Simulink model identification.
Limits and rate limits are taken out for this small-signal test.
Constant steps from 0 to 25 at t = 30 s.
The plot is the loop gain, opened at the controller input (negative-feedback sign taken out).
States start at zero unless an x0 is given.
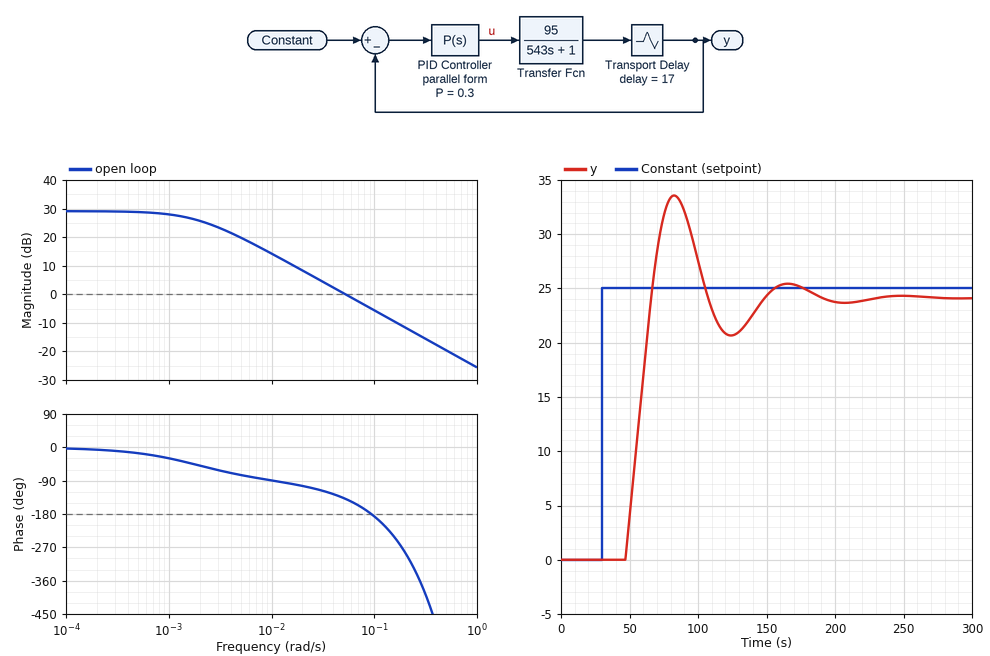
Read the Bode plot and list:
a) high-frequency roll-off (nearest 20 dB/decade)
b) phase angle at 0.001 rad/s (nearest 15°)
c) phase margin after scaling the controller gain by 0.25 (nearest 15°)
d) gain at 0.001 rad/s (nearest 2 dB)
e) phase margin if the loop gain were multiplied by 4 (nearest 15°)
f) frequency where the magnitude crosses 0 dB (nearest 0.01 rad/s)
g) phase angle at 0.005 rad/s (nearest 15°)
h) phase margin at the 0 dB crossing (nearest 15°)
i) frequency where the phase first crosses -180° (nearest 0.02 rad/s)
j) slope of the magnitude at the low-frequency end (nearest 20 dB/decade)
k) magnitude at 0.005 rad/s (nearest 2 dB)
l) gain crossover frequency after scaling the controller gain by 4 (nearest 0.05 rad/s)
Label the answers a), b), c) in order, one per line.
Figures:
a) -20 dB/decade
b) -30°
c) 90°
d) 28 dB
e) -120°
f) 0.05 rad/s
g) -75°
h) 45°
i) 0.10 rad/s
j) 0 dB/decade
k) 20 dB
l) 0.20 rad/s
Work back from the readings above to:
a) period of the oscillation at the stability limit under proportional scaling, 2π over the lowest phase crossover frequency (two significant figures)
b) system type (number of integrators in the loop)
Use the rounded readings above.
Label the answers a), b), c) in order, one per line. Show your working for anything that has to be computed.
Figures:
a) 2π / 0.1 = 63 s
b) 0
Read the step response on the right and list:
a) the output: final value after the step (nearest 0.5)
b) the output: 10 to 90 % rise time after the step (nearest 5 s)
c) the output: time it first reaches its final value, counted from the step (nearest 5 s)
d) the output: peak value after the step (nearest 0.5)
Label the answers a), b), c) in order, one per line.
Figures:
a) 24.0
b) 15 s
c) 35 s
d) 33.5
